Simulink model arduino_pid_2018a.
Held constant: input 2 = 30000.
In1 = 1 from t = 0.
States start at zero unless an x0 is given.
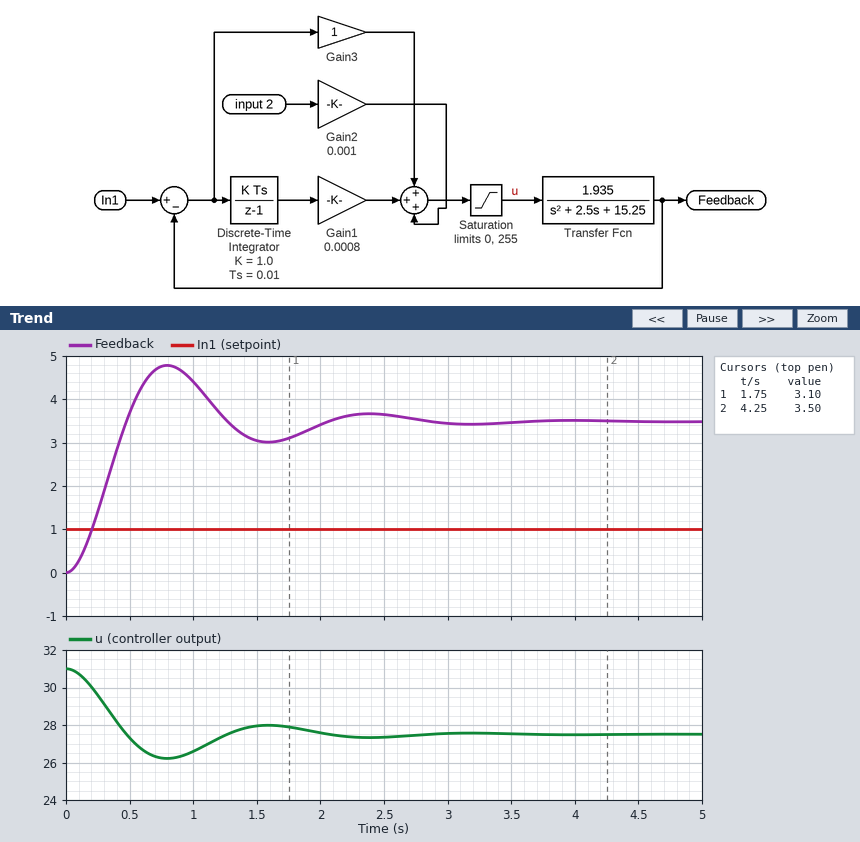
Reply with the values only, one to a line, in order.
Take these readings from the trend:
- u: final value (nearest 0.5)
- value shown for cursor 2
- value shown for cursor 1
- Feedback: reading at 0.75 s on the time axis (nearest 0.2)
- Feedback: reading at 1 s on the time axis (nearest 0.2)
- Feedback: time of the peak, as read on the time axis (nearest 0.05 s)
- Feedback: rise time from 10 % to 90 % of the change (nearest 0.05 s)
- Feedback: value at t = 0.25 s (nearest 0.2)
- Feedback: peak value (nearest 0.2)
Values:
27.5
3.50
3.10
4.8
4.4
0.80 s
0.30 s
1.4
4.8
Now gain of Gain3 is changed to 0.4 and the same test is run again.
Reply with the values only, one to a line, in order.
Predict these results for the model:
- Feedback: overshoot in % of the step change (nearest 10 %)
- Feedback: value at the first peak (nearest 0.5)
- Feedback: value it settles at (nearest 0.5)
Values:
40 %
5.0
3.5
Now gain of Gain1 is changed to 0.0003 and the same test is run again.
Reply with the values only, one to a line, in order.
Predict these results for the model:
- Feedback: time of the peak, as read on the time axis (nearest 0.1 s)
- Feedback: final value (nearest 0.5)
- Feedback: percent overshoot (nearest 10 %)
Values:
0.8 s
3.5
40 %
